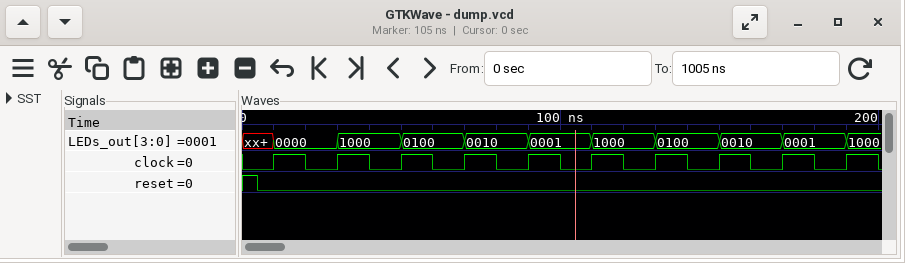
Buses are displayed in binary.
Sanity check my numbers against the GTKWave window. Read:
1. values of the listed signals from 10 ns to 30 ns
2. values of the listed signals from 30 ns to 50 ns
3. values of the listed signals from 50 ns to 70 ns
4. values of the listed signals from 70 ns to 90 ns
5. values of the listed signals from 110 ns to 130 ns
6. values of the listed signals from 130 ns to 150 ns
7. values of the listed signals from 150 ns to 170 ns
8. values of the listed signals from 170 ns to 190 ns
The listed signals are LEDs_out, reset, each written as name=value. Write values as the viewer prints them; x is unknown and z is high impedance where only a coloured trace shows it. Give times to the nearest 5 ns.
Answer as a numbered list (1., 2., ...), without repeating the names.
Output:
1. LEDs_out=0000, reset=0
2. LEDs_out=1000, reset=0
3. LEDs_out=0100, reset=0
4. LEDs_out=0010, reset=0
5. LEDs_out=1000, reset=0
6. LEDs_out=0100, reset=0
7. LEDs_out=0010, reset=0
8. LEDs_out=0001, reset=0
